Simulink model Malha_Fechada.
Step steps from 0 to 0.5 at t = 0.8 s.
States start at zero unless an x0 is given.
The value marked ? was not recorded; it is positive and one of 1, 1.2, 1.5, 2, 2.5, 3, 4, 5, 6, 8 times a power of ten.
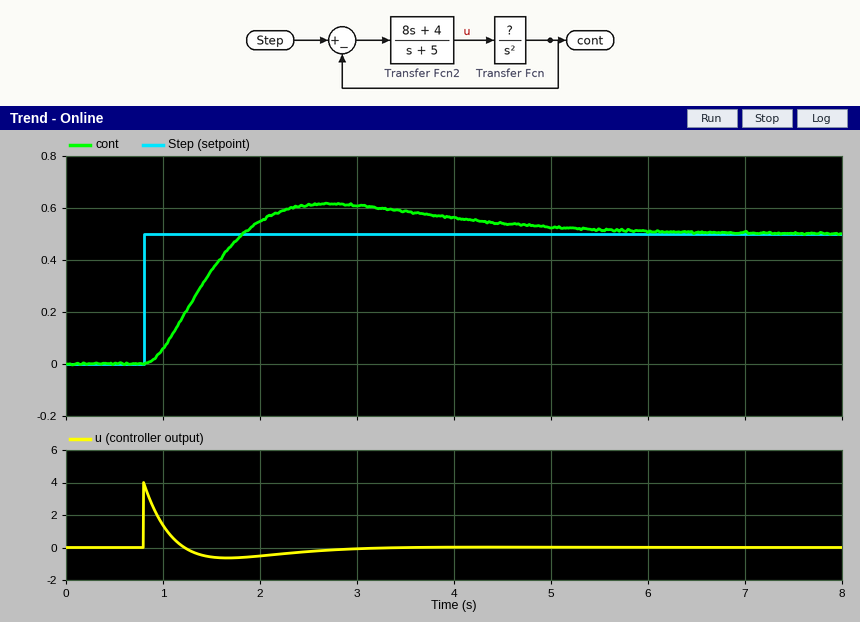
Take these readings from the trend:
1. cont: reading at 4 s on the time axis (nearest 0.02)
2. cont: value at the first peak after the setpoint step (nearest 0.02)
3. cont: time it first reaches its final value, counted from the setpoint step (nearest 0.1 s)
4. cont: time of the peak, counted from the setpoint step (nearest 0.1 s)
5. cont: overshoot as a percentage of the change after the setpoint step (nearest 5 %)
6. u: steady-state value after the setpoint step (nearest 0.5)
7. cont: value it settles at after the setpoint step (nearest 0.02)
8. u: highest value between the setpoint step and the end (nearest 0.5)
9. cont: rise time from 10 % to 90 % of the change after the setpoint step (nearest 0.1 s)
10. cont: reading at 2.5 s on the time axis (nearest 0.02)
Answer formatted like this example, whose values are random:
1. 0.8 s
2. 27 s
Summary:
1. 0.56
2. 0.62
3. 1.0 s
4. 1.9 s
5. 25 %
6. 0.0
7. 0.50
8. 4.0
9. 0.7 s
10. 0.62
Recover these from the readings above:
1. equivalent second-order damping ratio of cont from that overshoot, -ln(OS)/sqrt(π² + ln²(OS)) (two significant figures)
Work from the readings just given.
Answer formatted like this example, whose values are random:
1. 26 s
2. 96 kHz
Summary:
1. 0.40
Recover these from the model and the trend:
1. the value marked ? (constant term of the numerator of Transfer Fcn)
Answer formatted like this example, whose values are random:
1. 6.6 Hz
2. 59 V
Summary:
1. 1
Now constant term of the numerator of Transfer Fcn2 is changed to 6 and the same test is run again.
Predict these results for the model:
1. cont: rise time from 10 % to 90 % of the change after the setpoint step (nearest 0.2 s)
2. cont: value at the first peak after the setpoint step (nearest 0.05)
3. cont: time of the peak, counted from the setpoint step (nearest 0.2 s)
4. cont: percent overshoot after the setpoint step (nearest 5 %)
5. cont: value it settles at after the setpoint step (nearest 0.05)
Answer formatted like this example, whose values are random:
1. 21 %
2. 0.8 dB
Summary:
1. 0.6 s
2. 0.65
3. 1.8 s
4. 30 %
5. 0.50
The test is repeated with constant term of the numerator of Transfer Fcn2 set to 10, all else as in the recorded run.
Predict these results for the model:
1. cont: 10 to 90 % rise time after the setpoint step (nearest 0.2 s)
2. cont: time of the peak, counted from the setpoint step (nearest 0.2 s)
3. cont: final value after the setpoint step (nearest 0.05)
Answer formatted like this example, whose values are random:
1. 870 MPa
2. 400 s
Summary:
1. 0.6 s
2. 1.6 s
3. 0.50
